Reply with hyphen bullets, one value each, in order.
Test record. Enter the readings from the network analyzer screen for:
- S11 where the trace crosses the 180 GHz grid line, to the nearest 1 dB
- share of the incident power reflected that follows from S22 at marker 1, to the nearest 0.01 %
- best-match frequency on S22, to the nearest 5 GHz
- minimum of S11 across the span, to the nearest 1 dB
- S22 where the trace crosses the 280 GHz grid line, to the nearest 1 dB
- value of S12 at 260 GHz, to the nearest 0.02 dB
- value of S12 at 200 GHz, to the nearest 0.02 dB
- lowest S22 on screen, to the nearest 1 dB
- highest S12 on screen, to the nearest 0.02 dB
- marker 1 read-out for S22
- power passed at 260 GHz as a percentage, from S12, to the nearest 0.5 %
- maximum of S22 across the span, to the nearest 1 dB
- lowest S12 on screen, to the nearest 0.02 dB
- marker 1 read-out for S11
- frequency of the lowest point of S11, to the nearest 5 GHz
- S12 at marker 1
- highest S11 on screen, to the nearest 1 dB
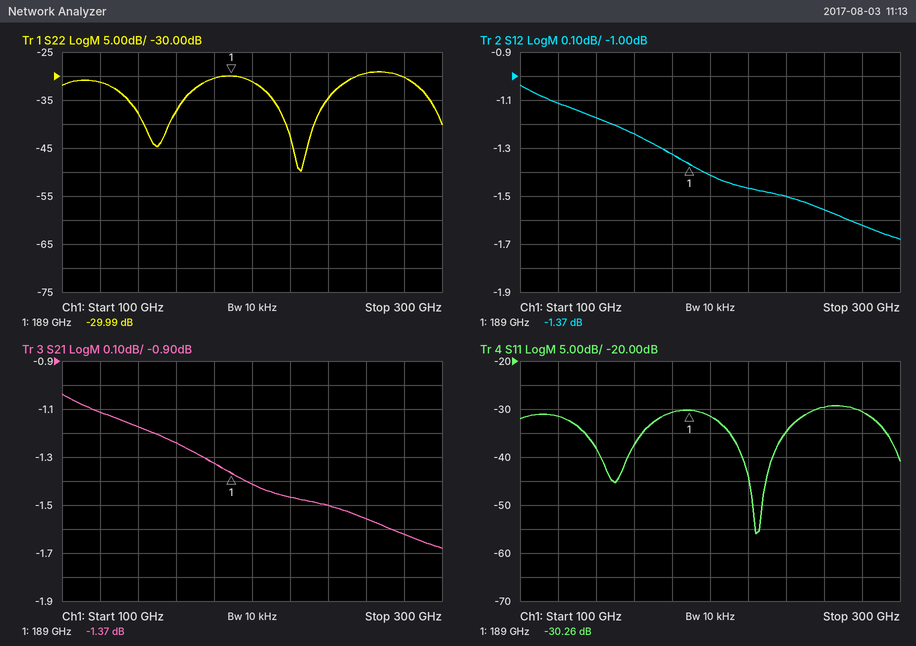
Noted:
- -31 dB
- 0.10 %
- 225 GHz
- -56 dB
- -30 dB
- -1.56 dB
- -1.42 dB
- -50 dB
- -1.04 dB
- -29.99 dB
- 70.0 %
- -29 dB
- -1.68 dB
- -30.26 dB
- 225 GHz
- -1.37 dB
- -29 dB
